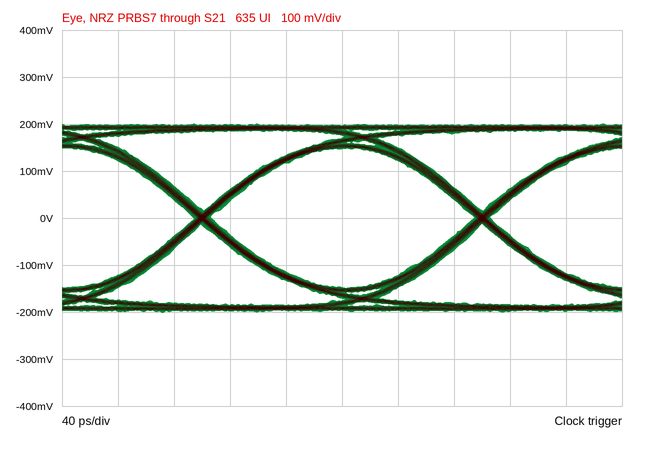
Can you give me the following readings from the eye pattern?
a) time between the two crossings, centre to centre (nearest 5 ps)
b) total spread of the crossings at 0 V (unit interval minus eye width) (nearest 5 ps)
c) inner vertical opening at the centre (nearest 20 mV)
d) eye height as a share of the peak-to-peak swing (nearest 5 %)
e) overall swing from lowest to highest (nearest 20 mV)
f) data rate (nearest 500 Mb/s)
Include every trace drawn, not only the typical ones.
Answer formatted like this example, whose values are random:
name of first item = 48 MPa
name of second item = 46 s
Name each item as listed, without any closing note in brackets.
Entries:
time between the two crossings, centre to centre = 200 ps
total spread of the crossings at 0 V (unit interval minus eye width) = 10 ps
inner vertical opening at the centre = 300 mV
eye height as a share of the peak-to-peak swing = 75 %
overall swing from lowest to highest = 400 mV
data rate = 5.0 Gb/s
